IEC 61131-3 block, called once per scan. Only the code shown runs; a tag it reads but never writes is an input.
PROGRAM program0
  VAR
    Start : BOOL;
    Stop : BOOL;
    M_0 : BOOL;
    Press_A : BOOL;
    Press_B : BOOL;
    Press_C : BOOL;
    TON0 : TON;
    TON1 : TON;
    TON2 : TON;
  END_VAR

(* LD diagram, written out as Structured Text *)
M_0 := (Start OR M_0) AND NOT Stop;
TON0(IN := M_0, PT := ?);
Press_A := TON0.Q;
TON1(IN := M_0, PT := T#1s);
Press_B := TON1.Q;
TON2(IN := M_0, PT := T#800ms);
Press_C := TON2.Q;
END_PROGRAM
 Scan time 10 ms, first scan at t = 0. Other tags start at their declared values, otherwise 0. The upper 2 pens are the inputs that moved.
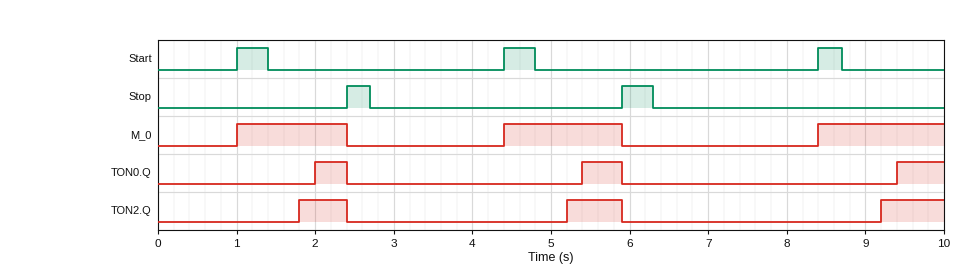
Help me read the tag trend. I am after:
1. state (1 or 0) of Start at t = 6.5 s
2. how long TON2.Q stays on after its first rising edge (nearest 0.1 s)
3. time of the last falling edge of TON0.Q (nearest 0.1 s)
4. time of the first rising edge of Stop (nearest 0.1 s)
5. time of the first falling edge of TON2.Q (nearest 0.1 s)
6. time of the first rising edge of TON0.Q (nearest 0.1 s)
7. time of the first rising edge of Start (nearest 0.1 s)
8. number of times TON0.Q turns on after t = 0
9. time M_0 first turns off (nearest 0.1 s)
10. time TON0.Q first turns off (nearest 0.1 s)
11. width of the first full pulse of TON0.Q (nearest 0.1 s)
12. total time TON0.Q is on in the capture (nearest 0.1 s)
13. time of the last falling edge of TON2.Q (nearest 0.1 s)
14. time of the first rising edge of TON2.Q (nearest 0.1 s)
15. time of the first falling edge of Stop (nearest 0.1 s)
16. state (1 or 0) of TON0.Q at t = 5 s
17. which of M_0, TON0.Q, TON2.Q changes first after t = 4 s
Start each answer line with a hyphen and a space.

- 0
- 0.6 s
- 5.9 s
- 2.4 s
- 2.4 s
- 2.0 s
- 1.0 s
- 3
- 2.4 s
- 2.4 s
- 0.4 s
- 1.5 s
- 5.9 s
- 1.8 s
- 2.7 s
- 0
- M_0
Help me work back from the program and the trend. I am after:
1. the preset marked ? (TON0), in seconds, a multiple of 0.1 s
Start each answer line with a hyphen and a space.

- 1.0 s
